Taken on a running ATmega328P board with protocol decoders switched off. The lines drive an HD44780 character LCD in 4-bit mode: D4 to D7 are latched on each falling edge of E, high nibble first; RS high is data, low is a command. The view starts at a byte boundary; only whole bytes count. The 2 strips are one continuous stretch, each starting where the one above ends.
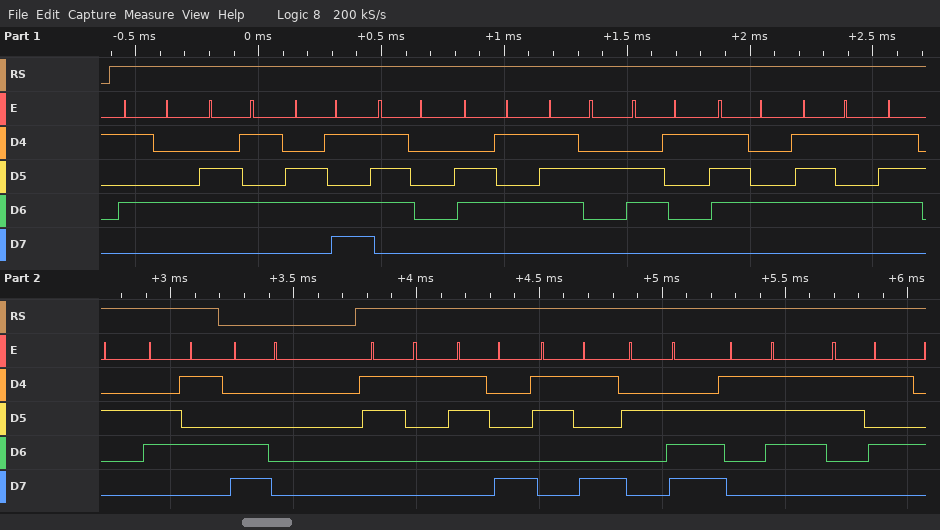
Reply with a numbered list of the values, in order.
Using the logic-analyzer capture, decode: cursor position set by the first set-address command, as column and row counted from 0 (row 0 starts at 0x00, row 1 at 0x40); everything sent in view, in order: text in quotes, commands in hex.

1. column 0, row 1
2. "Temperature" 0xC0 "189.75"
